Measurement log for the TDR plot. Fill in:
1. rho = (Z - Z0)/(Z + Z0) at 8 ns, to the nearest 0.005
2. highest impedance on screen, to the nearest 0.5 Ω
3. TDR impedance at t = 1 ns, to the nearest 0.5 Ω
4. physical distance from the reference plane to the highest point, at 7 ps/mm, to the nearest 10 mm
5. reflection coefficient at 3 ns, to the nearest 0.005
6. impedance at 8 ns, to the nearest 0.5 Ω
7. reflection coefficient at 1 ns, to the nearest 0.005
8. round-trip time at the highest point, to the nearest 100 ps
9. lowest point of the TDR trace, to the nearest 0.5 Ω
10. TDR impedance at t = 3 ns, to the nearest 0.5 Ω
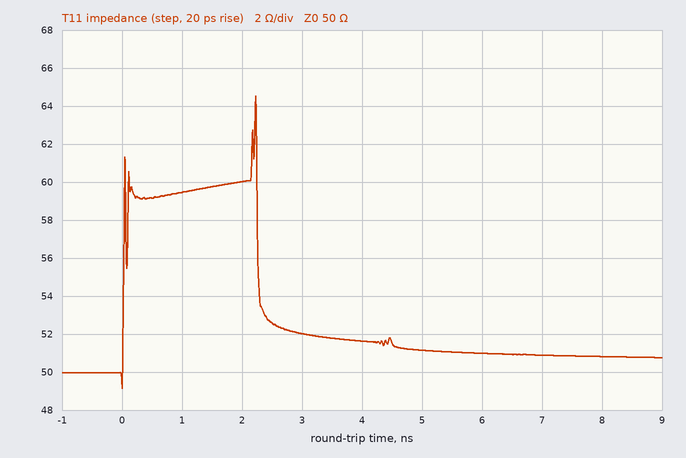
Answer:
+0.010
64.5 Ω
59.5 Ω
160 mm
+0.020
51.0 Ω
+0.085
2.2 ns
49.0 Ω
52.0 Ω
